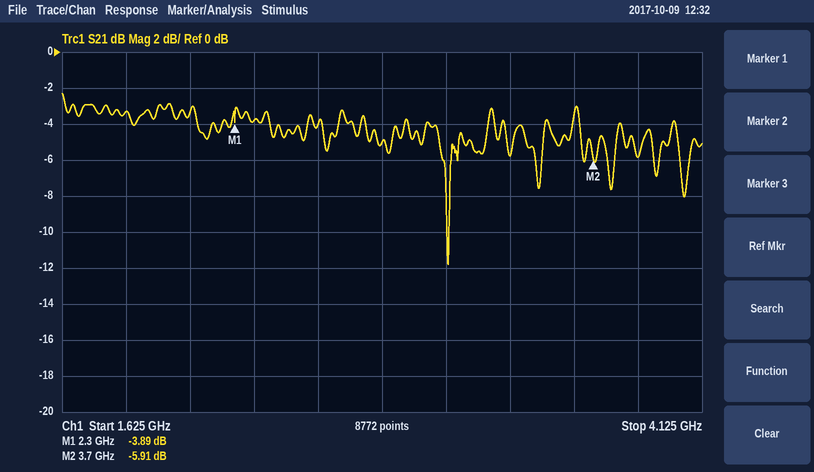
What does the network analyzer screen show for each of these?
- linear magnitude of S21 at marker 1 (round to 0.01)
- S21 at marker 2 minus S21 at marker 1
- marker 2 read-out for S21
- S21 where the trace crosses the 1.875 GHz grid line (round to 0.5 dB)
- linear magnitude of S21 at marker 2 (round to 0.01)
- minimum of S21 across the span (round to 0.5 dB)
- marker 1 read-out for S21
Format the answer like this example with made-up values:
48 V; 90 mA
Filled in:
0.64; -2.02 dB; -5.91 dB; -3.5 dB; 0.51; -12.0 dB; -3.89 dB
